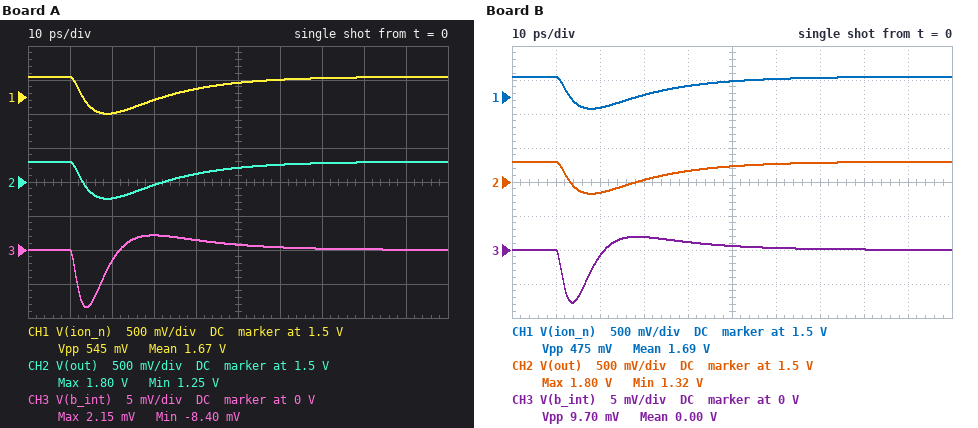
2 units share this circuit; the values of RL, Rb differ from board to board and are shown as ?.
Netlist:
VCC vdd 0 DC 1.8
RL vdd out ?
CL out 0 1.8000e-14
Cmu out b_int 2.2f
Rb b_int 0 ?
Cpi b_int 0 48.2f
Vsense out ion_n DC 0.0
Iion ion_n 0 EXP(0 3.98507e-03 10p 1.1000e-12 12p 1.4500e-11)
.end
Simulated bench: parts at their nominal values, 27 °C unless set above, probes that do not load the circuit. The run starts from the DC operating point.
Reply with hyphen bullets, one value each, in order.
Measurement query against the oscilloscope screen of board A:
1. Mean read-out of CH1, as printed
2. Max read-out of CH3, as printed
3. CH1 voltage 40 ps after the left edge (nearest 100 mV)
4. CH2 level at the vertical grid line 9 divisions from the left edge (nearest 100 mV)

- 1.67 V
- 2.15 mV
- 1.6 V
- 1.8 V
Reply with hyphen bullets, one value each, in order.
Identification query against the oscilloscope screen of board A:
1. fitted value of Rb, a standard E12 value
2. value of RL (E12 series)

- 47 Ω
- 220 Ω
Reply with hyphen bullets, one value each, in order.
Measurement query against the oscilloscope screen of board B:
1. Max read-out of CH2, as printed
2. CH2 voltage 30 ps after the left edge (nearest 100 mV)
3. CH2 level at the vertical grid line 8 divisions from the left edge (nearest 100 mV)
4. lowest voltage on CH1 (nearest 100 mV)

- 1.80 V
- 1.5 V
- 1.8 V
- 1.3 V
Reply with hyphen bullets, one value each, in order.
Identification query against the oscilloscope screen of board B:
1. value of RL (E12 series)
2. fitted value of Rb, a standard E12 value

- 180 Ω
- 47 Ω
